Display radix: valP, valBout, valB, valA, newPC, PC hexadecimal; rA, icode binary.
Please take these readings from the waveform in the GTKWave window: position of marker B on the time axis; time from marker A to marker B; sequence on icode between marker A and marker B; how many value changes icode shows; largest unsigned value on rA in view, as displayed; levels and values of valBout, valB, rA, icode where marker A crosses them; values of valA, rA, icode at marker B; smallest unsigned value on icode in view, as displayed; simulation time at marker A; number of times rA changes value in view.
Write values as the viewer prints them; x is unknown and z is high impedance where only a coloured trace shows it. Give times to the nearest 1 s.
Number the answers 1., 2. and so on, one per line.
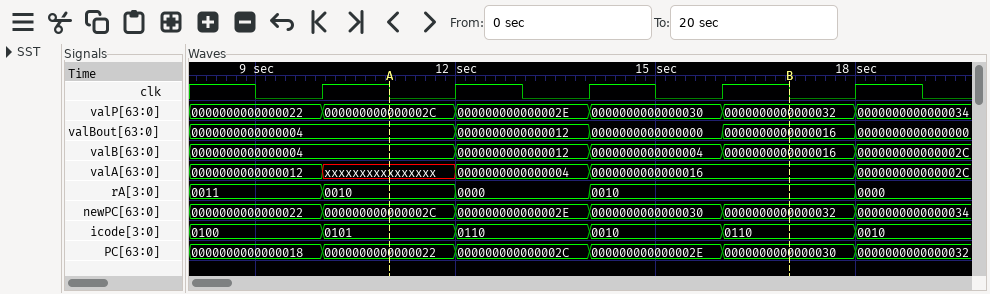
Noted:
1. 17 s
2. 6 s
3. 0101, 0110, 0010, 0110
4. 5
5. 0011
6. valBout=0000000000000004, valB=0000000000000004, rA=0010, icode=0101
7. valA=0000000000000016, rA=0010, icode=0110
8. 0010
9. 11 s
10. 4
